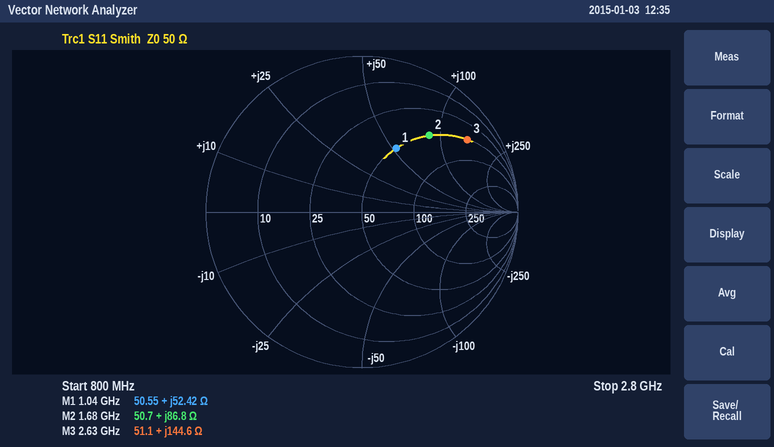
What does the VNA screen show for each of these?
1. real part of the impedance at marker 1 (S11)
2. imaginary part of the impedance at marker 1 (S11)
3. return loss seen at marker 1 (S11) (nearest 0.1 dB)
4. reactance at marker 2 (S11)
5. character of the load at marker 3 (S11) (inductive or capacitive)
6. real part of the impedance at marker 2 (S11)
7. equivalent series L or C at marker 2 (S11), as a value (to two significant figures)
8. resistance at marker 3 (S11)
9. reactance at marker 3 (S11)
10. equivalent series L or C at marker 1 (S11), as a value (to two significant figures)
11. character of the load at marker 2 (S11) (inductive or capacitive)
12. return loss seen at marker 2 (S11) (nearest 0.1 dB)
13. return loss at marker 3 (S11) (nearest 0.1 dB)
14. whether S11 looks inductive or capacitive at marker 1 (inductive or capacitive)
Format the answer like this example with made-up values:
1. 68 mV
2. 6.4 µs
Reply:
1. 50.55 Ω
2. +52.42 Ω
3. 6.7 dB
4. +86.8 Ω
5. inductive
6. 50.7 Ω
7. 8.2 nH
8. 51.1 Ω
9. +144.6 Ω
10. 8.0 nH
11. inductive
12. 3.7 dB
13. 1.7 dB
14. inductive
